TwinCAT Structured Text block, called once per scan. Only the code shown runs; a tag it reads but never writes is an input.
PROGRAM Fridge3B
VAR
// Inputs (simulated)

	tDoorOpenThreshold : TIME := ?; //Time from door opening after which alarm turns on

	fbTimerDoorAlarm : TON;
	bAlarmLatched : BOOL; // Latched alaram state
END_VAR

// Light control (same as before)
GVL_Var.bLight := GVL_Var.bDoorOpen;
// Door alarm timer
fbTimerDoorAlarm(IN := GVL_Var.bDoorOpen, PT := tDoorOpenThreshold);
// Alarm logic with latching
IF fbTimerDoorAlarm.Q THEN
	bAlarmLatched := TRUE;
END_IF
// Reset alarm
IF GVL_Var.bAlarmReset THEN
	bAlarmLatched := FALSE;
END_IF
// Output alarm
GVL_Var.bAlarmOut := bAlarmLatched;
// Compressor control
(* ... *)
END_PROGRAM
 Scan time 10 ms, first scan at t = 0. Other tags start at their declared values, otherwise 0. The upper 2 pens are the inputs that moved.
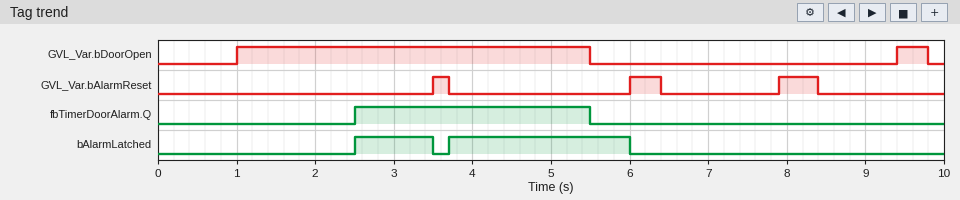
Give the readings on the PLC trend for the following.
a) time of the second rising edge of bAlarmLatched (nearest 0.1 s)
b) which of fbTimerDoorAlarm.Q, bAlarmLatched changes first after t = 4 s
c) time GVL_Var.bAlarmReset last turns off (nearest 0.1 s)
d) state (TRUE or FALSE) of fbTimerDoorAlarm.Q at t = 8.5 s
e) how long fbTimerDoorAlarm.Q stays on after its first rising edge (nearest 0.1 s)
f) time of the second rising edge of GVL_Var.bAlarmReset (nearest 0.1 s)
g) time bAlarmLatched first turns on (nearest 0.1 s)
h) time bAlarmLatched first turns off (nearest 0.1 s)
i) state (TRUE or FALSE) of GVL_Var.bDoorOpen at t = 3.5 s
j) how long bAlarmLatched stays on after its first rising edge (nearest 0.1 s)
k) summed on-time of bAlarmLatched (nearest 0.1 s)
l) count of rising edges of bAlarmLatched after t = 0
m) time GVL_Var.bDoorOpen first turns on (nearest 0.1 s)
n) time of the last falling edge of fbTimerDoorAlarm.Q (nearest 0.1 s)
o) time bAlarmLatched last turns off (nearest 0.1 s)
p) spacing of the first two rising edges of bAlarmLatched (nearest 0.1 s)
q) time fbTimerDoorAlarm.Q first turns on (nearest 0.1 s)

3.7 s
fbTimerDoorAlarm.Q
8.4 s
FALSE
3.0 s
6.0 s
2.5 s
3.5 s
TRUE
1.0 s
3.3 s
2
1.0 s
5.5 s
6.0 s
1.2 s
2.5 s
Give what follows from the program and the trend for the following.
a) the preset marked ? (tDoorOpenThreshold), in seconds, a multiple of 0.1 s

1.5 s
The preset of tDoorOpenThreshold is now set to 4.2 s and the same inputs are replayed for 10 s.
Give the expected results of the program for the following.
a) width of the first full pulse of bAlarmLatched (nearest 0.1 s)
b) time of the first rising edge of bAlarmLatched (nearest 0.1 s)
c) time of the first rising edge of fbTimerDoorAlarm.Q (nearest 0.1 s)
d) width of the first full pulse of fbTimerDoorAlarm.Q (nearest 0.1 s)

0.8 s
5.2 s
5.2 s
0.3 s
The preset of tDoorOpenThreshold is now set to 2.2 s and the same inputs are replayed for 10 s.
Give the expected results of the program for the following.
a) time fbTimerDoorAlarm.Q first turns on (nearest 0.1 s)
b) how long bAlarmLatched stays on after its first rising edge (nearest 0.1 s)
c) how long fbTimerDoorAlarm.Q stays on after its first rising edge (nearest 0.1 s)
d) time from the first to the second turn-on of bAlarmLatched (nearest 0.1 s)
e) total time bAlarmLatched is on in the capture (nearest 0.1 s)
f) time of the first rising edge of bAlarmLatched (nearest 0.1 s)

3.2 s
0.3 s
2.3 s
0.5 s
2.6 s
3.2 s
